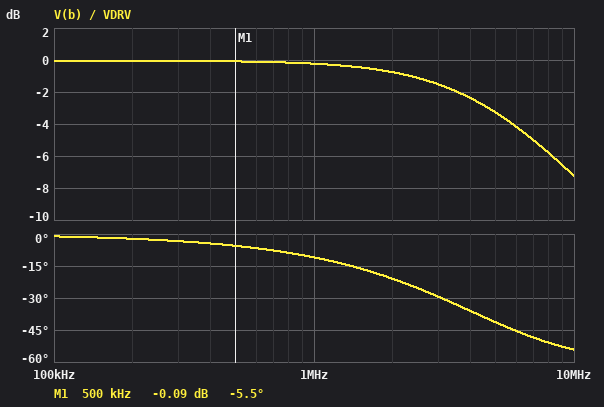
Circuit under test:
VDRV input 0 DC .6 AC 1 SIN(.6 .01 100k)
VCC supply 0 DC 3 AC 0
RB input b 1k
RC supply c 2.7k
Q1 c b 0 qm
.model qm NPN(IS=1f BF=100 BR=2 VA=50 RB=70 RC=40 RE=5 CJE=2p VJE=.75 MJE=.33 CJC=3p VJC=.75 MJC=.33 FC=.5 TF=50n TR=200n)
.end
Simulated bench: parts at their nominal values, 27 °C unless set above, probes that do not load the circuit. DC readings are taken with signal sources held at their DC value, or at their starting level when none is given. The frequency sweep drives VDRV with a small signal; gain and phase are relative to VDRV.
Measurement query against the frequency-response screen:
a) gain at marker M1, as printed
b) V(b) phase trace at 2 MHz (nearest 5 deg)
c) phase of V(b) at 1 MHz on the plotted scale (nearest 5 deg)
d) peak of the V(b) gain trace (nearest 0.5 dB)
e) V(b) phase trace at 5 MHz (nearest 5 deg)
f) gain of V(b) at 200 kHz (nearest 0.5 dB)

-0.09 dB
-20 deg
-10 deg
0 dB
-40 deg
0 dB
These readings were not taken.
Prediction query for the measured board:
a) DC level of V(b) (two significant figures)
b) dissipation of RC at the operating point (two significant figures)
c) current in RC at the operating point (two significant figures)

600 mV
410 nW
12 µA
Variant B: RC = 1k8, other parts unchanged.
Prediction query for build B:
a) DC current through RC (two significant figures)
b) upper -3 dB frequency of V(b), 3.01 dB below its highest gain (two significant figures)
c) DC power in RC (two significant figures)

12 µA
4.9 MHz
270 nW
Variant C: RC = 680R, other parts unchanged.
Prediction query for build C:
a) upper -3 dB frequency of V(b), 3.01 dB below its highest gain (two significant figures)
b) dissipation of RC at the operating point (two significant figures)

5.1 MHz
100 nW
